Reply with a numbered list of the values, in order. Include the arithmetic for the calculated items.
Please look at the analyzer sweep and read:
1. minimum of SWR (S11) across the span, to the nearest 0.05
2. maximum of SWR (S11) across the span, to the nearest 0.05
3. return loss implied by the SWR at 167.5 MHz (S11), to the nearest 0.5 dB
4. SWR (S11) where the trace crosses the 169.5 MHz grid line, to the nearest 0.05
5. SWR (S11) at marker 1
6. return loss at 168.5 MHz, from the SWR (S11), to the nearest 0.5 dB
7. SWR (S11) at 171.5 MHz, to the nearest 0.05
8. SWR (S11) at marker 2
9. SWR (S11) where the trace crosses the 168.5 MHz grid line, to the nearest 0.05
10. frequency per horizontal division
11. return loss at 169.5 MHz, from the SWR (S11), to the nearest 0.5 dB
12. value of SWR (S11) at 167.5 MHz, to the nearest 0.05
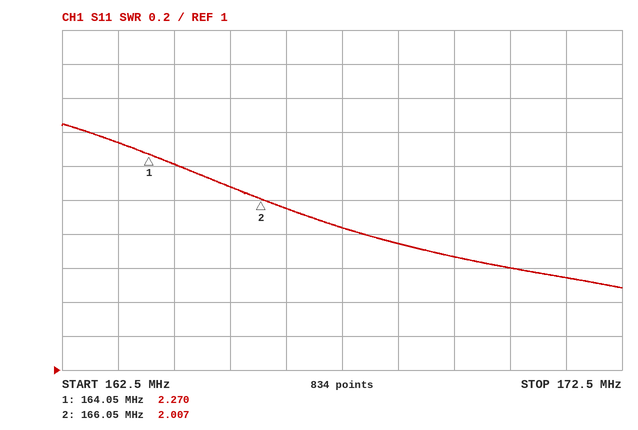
1. 1.50
2. 2.45
3. −20 log10((1.85 − 1)/(1.85 + 1)) ≈ 10.5 dB
4. 1.65
5. 2.270
6. −20 log10((1.75 − 1)/(1.75 + 1)) ≈ 11.3 dB, so 11.5 dB to the nearest 0.5 dB
7. 1.55
8. 2.007
9. 1.75
10. 1 MHz
11. −20 log10((1.65 − 1)/(1.65 + 1)) ≈ 12.2 dB, so 12.0 dB to the nearest 0.5 dB
12. 1.85
